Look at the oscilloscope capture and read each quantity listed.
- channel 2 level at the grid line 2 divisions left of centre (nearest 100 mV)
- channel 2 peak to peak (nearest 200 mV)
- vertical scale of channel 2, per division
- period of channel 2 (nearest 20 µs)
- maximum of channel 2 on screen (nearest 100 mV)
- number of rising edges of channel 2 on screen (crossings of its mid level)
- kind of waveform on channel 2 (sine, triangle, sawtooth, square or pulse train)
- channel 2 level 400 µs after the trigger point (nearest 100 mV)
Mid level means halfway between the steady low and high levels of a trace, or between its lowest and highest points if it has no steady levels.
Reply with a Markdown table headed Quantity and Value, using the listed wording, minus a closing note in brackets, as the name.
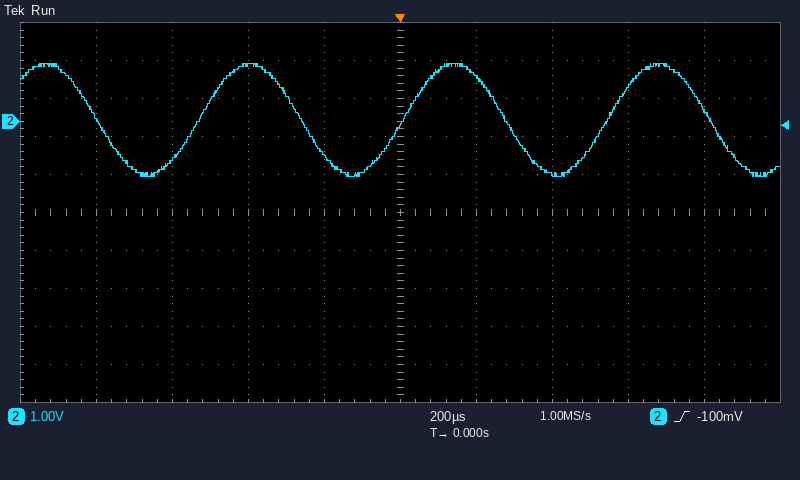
| Quantity | Value |
|---|---|
| channel 2 level at the grid line 2 divisions left of centre | 1.5 V |
| channel 2 peak to peak | 3.0 V |
| vertical scale of channel 2, per division | 1 V |
| period of channel 2 | 540 µs |
| maximum of channel 2 on screen | 1.5 V |
| number of rising edges of channel 2 on screen | 3 |
| kind of waveform on channel 2 | sine |
| channel 2 level 400 µs after the trigger point | -1.4 V |
